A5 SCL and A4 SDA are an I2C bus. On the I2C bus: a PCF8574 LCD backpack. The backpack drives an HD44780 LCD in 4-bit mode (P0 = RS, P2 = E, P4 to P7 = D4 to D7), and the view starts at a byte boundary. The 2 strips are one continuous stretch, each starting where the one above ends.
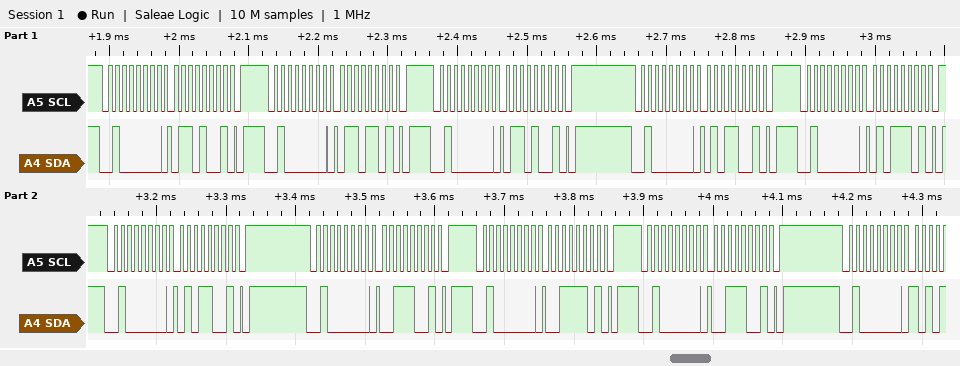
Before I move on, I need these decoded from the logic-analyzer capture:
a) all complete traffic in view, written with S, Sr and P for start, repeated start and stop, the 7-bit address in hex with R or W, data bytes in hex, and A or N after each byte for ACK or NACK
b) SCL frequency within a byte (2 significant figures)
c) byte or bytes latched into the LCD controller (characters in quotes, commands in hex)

S 20W A 69 A P S 20W A 6D A P S 20W A 69 A P S 20W A 59 A P S 20W A 5D A P S 20W A 59 A P S 20W A 39 A P S 20W A 3D A P S 20W A 39 A P S 20W A
100 kHz
'e'
